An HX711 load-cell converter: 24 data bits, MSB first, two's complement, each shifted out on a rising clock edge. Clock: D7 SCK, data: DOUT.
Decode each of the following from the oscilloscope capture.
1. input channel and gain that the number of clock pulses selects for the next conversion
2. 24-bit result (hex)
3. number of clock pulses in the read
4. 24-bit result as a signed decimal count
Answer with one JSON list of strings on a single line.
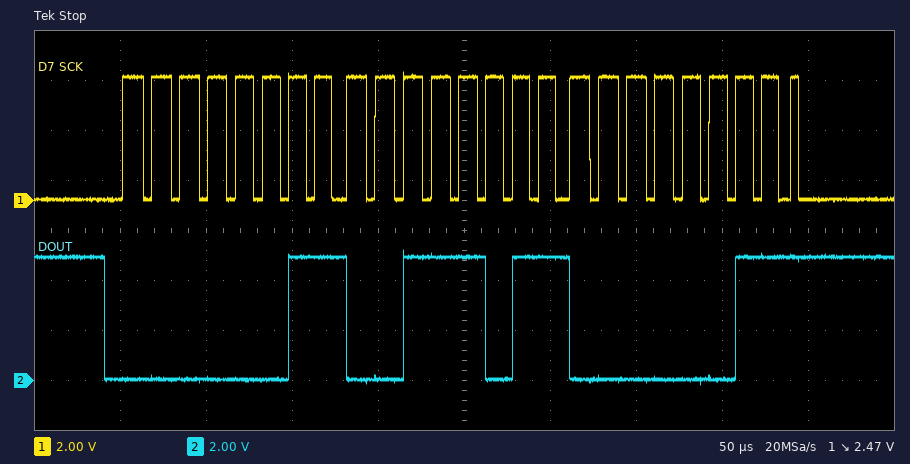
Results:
["channel A, gain 128", "0x033B03", "25", "211715"]
